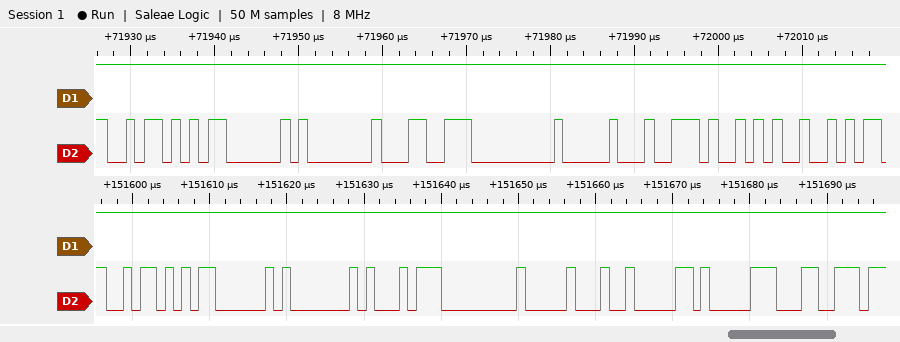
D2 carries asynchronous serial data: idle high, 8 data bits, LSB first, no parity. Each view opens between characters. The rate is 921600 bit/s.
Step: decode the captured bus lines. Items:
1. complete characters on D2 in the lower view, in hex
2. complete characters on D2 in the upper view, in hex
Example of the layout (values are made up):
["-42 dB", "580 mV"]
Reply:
["5A, 03, 01, D1, 00, 10, 82, C1, CC", "5A, 03, 01, CC, 00, 10, 2E, 25"]
